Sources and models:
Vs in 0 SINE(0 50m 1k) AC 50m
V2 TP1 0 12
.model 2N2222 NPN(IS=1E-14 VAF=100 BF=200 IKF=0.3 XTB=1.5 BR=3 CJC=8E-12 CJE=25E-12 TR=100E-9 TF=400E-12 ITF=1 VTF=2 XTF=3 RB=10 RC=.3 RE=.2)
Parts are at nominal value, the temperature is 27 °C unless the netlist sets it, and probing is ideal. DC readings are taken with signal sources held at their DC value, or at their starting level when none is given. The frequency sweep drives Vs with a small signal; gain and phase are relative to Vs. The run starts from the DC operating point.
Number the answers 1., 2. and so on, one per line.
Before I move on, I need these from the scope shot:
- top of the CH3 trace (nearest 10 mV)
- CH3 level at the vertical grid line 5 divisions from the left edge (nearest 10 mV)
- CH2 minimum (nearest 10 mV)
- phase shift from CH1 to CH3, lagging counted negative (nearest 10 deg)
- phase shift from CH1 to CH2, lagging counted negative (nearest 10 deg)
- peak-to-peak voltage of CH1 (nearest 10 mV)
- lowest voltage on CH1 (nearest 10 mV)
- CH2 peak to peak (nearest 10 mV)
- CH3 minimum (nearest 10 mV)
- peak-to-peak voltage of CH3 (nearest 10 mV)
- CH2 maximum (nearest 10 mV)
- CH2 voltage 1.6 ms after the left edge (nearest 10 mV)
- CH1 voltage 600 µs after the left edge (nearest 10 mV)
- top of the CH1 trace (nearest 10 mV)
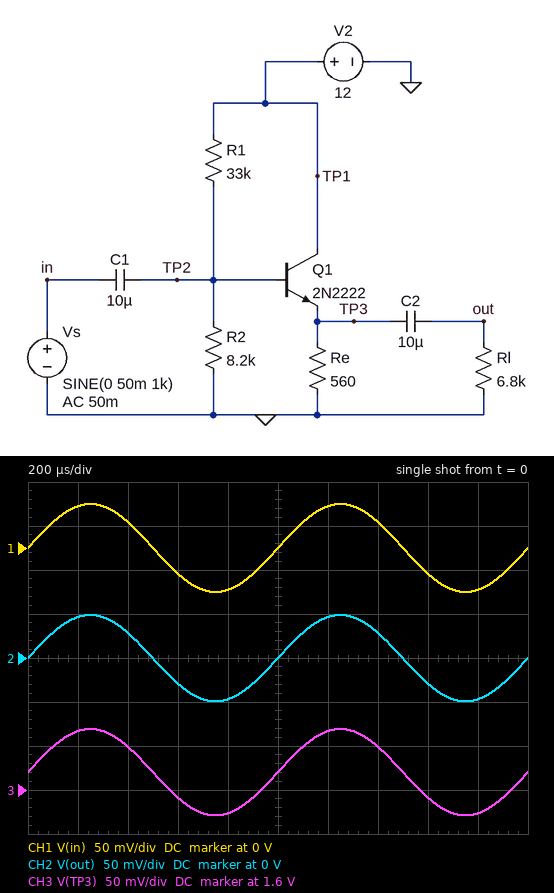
1. 1.67 V
2. 1.62 V
3. -50 mV
4. 0 deg
5. 0 deg
6. 100 mV
7. -50 mV
8. 100 mV
9. 1.57 V
10. 100 mV
11. 50 mV
12. -30 mV
13. -30 mV
14. 50 mV
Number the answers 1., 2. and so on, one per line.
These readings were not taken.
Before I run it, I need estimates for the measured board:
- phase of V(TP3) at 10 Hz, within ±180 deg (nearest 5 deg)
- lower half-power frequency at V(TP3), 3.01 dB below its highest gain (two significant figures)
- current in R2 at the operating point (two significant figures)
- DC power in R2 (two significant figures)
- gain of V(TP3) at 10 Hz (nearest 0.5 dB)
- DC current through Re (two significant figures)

1. 15 deg
2. 2.6 Hz
3. 280 µA
4. 650 µW
5. -0.5 dB
6. 2.9 mA
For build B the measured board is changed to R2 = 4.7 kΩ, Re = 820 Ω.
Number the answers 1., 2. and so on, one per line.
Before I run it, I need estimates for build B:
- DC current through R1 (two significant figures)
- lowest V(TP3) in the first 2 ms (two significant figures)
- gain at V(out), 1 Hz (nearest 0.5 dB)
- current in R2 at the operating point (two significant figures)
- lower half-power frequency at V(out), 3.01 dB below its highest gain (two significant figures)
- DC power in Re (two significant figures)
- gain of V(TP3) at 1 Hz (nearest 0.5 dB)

1. 320 µA
2. 780 mV
3. -20.5 dB
4. 310 µA
5. 5.0 Hz
6. 830 µW
7. -12.5 dB
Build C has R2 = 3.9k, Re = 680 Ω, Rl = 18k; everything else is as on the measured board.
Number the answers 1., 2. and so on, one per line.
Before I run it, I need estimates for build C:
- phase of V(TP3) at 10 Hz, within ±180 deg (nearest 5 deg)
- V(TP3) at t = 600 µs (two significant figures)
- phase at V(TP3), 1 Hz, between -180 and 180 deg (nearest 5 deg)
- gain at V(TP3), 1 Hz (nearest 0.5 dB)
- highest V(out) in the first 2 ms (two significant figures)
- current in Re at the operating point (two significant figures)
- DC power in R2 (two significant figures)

1. 25 deg
2. 580 mV
3. 80 deg
4. -14.0 dB
5. 48 mV
6. 890 µA
7. 400 µW
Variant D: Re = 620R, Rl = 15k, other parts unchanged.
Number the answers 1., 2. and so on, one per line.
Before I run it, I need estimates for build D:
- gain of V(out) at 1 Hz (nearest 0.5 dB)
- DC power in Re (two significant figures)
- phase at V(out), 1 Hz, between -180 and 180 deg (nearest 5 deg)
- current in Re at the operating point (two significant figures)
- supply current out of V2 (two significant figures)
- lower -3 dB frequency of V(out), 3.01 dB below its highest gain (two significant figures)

1. -12.0 dB
2. 4.3 mW
3. 115 deg
4. 2.6 mA
5. 2.9 mA
6. 2.9 Hz
